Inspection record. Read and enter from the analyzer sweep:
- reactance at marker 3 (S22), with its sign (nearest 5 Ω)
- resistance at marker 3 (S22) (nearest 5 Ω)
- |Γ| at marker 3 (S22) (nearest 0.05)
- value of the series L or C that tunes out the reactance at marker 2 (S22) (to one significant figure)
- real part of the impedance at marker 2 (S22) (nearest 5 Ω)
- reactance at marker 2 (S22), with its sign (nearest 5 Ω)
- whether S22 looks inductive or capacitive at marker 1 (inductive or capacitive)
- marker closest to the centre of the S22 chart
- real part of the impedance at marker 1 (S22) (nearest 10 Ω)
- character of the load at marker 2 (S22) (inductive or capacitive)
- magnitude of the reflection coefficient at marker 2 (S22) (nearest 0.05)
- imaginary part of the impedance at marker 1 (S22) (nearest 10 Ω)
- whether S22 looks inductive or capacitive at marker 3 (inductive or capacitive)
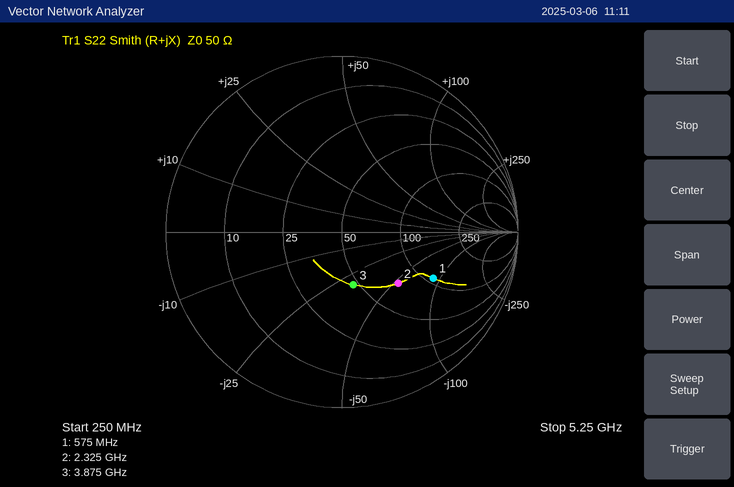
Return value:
-30 Ω
45 Ω
0.30
4 nH
75 Ω
-55 Ω
capacitive
marker 3
110 Ω
capacitive
0.45
-90 Ω
capacitive
